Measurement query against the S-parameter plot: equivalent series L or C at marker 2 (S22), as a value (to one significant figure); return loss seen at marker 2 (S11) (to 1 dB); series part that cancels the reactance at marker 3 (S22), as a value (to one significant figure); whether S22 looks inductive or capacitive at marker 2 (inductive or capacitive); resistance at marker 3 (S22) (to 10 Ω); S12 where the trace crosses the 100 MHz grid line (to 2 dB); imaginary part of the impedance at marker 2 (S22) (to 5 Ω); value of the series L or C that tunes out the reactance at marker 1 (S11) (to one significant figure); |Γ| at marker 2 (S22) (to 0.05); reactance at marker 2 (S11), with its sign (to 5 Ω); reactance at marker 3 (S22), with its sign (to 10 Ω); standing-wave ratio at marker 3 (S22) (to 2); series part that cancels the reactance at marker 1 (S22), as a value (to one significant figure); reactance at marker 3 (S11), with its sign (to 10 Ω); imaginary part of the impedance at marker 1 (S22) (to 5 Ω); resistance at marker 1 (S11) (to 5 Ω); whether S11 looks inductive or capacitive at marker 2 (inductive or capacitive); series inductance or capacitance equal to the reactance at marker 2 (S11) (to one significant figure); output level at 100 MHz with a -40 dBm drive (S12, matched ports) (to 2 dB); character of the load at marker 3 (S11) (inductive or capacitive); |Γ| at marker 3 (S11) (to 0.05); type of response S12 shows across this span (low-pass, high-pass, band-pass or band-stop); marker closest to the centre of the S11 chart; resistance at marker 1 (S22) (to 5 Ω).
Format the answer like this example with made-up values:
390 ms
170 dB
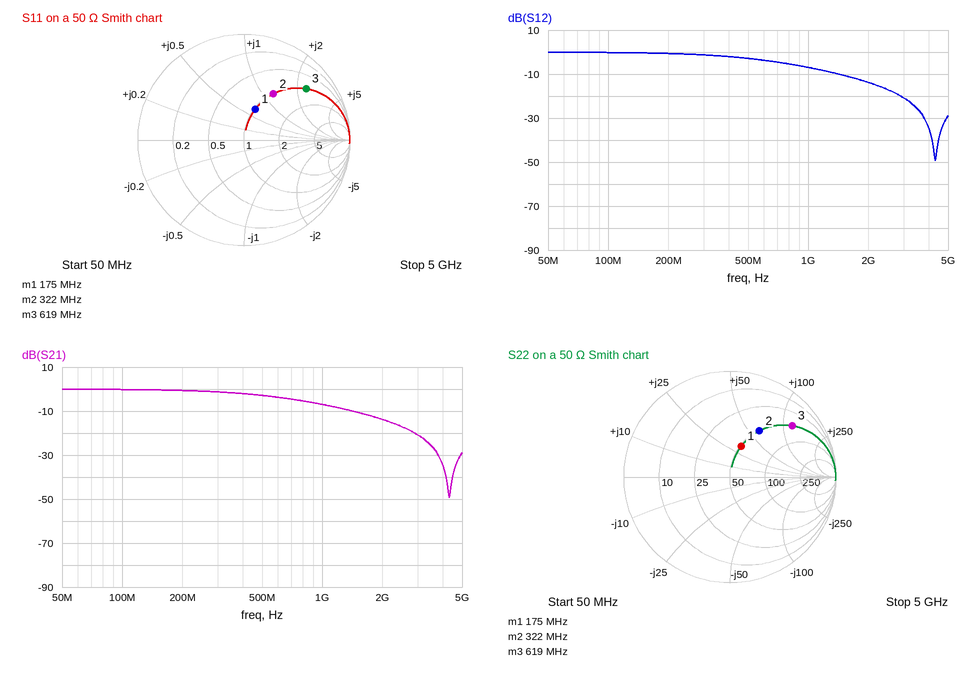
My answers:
30 nH
6 dB
2 pF
inductive
50 Ω
0 dB
+60 Ω
30 pF
0.50
+60 Ω
+120 Ω
8
30 pF
+120 Ω
+35 Ω
50 Ω
inductive
30 nH
-40 dBm
inductive
0.75
low-pass
marker 1
50 Ω
